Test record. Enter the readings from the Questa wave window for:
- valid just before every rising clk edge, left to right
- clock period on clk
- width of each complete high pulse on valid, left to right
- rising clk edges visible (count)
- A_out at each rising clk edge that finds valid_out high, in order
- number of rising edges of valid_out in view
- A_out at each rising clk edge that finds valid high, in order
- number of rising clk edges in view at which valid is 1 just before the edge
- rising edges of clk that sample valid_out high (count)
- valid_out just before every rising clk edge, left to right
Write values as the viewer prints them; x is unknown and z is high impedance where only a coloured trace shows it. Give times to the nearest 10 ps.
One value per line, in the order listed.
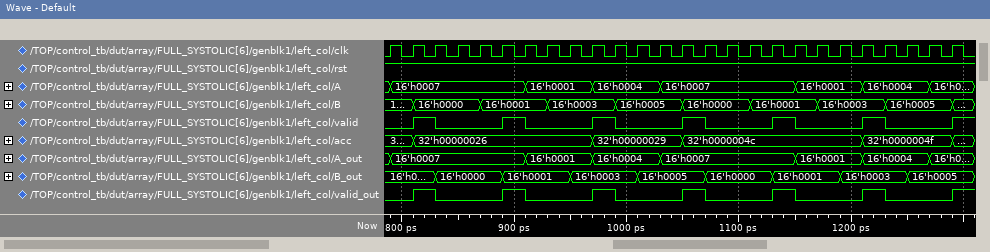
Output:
0 0 1 0 0 0 1 0 0 0 1 0 0 0 1 0 0 0 1 0 0 0 1 0 0 0
20 ps
20 ps, 20 ps, 20 ps, 20 ps, 20 ps, 20 ps
26
16'h0007, 16'h0007, 16'h0004, 16'h0007, 16'h0007, 16'h0004
7
16'h0007, 16'h0007, 16'h0004, 16'h0007, 16'h0007, 16'h0004
6
6
0 0 1 0 0 0 1 0 0 0 1 0 0 0 1 0 0 0 1 0 0 0 1 0 0 0
